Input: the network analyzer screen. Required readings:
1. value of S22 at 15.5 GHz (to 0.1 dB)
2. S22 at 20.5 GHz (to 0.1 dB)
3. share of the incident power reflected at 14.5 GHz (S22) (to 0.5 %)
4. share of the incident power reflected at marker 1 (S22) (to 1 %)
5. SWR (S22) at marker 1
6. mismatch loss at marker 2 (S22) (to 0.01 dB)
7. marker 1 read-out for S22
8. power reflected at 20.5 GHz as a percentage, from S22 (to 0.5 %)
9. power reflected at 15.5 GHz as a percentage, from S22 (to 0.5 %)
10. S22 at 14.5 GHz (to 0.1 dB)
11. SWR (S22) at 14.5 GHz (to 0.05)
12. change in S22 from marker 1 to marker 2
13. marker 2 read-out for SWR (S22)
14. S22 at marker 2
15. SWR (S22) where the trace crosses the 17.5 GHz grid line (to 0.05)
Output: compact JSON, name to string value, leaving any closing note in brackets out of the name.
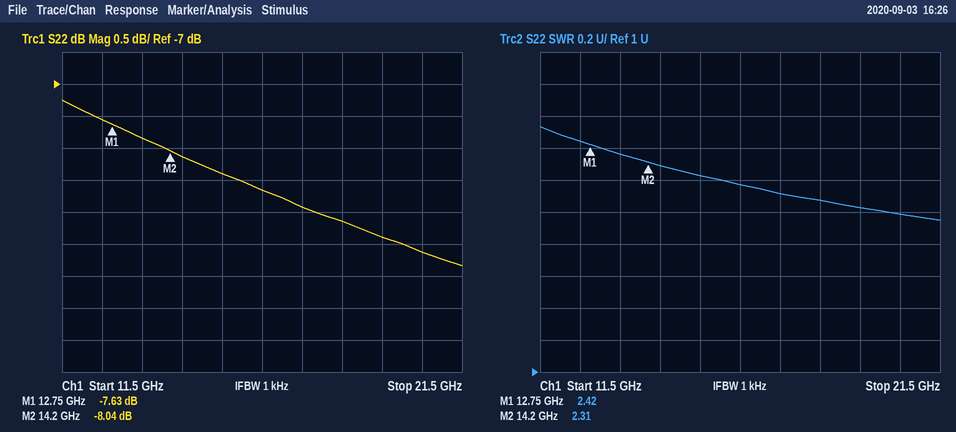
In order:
{"value of S22 at 15.5 GHz": "-8.4 dB", "S22 at 20.5 GHz": "-9.6 dB", "share of the incident power reflected at 14.5 GHz (S22)": "15.5 %", "share of the incident power reflected at marker 1 (S22)": "17 %", "SWR (S22) at marker 1": "2.42", "mismatch loss at marker 2 (S22)": "0.74 dB", "marker 1 read-out for S22": "-7.63 dB", "power reflected at 20.5 GHz as a percentage, from S22": "11.0 %", "power reflected at 15.5 GHz as a percentage, from S22": "14.5 %", "S22 at 14.5 GHz": "-8.1 dB", "SWR (S22) at 14.5 GHz": "2.30", "change in S22 from marker 1 to marker 2": "-0.41 dB", "marker 2 read-out for SWR": "2.31", "S22 at marker 2": "-8.04 dB", "SWR (S22) where the trace crosses the 17.5 GHz grid line": "2.10"}
